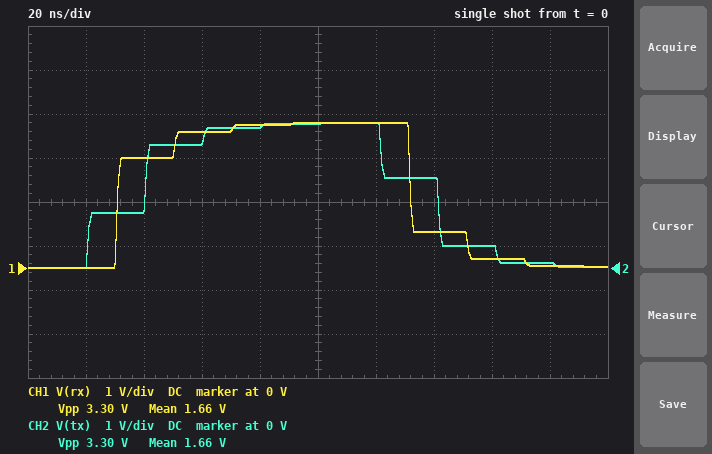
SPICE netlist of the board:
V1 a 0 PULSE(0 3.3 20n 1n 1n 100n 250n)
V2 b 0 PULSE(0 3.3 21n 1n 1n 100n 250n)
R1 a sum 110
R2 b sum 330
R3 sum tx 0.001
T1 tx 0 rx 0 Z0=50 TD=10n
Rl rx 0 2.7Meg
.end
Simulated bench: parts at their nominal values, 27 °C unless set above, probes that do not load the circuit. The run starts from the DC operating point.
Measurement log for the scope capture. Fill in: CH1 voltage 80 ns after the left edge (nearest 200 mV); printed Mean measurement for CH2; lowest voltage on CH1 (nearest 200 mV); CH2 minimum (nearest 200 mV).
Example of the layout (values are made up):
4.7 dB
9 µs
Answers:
3.2 V
1.66 V
0 V
0 V
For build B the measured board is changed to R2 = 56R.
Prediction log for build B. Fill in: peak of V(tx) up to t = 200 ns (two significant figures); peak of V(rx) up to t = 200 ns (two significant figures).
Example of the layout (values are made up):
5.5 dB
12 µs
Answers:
3.5 V
3.8 V
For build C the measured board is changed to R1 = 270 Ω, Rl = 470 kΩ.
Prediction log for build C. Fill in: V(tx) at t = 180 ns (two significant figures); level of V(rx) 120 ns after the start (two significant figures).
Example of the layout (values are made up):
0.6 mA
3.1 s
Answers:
590 mV
3.2 V
